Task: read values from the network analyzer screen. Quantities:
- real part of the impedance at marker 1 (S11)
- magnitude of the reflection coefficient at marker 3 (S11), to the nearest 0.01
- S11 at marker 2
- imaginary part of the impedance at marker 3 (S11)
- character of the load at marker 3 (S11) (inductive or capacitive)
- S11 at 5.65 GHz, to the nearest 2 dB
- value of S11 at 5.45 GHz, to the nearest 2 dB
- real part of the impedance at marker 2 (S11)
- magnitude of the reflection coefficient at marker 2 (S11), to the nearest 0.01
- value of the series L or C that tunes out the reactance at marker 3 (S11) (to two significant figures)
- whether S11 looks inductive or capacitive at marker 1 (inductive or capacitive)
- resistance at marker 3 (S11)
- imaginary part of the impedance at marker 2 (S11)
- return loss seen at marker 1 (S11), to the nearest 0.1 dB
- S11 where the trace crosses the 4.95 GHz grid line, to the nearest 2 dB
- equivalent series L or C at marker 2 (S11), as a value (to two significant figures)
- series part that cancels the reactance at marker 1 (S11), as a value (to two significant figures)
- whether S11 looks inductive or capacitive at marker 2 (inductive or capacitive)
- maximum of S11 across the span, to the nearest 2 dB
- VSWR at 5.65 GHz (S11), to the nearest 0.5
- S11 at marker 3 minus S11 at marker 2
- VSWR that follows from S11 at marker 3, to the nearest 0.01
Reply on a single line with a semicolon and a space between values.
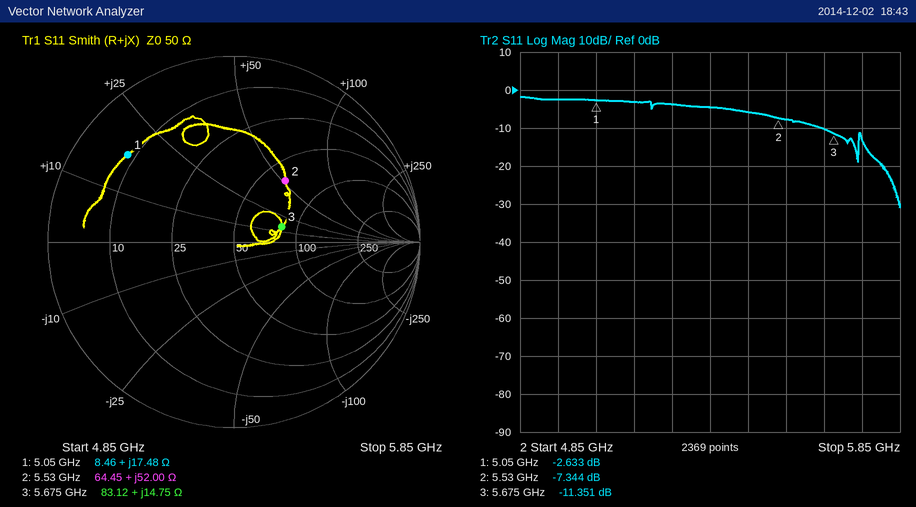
8.46 Ω; 0.27; -7.344 dB; +14.75 Ω; inductive; -10 dB; -6 dB; 64.45 Ω; 0.43; 1.9 pF; inductive; 83.12 Ω; +52.00 Ω; 2.6 dB; -2 dB; 1.5 nH; 1.8 pF; inductive; -2 dB; 2.0; -4.007 dB; 1.74
